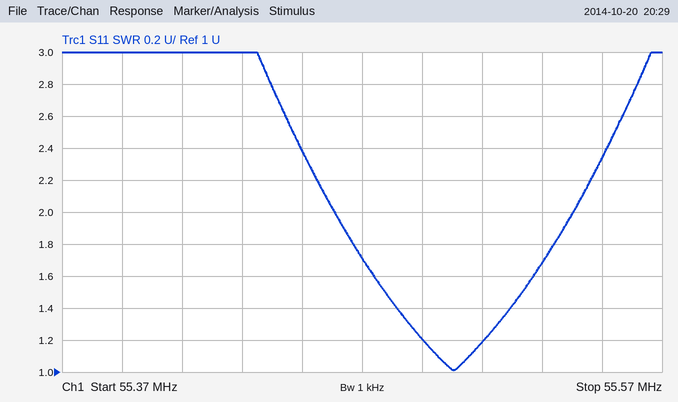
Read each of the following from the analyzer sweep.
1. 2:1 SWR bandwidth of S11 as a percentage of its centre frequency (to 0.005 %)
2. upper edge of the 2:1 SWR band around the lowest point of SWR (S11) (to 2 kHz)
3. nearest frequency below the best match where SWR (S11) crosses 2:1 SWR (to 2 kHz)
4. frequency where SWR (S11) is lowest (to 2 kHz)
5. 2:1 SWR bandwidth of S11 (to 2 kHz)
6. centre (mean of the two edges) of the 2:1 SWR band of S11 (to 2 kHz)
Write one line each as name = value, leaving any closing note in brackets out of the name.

2:1 SWR bandwidth of S11 as a percentage of its centre frequency = 0.145 %
upper edge of the 2:1 SWR band around the lowest point of SWR (S11) = 55.540 MHz
nearest frequency below the best match where SWR (S11) crosses 2:1 SWR = 55.460 MHz
frequency where SWR (S11) is lowest = 55.500 MHz
2:1 SWR bandwidth of S11 = 80 kHz
centre (mean of the two edges) of the 2:1 SWR band of S11 = 55.500 MHz
